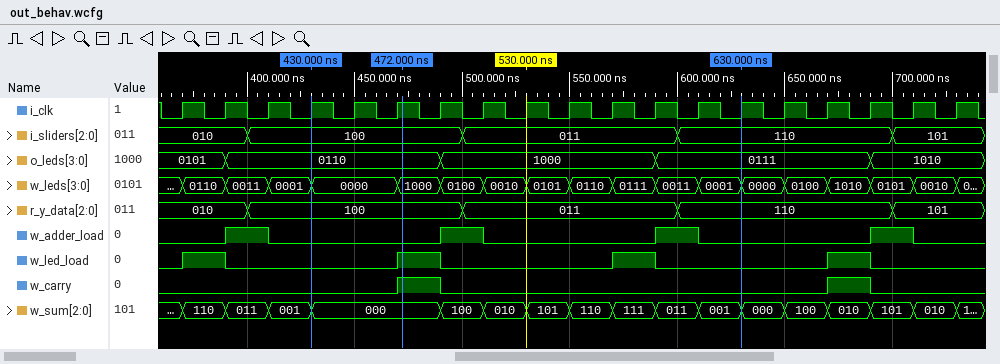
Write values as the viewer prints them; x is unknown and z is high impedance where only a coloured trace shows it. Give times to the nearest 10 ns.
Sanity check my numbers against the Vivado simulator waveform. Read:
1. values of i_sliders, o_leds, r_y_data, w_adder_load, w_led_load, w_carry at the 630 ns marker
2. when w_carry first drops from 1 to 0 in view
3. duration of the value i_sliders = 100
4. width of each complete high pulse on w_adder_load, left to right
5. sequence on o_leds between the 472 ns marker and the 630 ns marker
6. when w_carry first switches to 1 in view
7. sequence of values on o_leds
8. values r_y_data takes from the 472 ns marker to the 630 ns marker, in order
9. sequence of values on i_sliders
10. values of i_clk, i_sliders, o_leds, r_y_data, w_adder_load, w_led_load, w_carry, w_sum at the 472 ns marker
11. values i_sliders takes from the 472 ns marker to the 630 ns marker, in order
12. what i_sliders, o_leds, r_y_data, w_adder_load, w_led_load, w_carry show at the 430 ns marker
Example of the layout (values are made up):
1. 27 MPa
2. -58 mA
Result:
1. i_sliders=110, o_leds=0111, r_y_data=110, w_adder_load=0, w_led_load=0, w_carry=0
2. 490 ns
3. 100 ns
4. 20 ns, 20 ns, 20 ns, 20 ns
5. 0110, 1000, 0111
6. 470 ns
7. 0101, 0110, 1000, 0111, 1010
8. 100, 011, 110
9. 010, 100, 011, 110, 101
10. i_clk=1, i_sliders=100, o_leds=0110, r_y_data=100, w_adder_load=0, w_led_load=1, w_carry=1, w_sum=000
11. 100, 011, 110
12. i_sliders=100, o_leds=0110, r_y_data=100, w_adder_load=0, w_led_load=0, w_carry=0
